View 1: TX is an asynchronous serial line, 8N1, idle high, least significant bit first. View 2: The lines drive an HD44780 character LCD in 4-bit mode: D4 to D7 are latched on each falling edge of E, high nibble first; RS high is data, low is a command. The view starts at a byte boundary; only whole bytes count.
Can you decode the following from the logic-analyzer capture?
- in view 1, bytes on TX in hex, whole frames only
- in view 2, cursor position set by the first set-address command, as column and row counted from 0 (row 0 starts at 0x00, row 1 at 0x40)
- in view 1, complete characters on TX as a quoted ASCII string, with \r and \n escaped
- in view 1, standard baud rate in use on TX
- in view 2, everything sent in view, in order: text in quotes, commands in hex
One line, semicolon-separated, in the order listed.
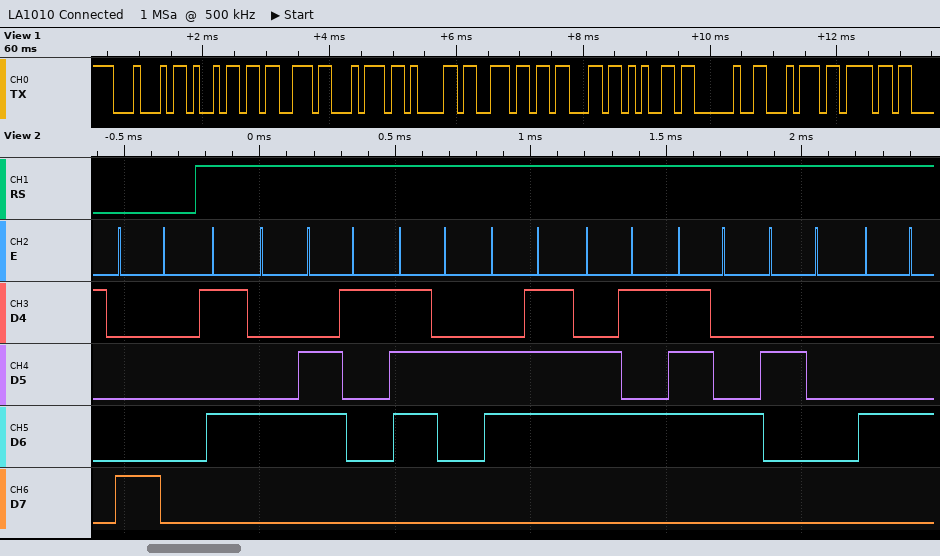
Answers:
44 69 73 74 61 6E 63 65 20 74 6F; column 0, row 0; "Distance to"; 9600 baud; 0x80 "Target D"
